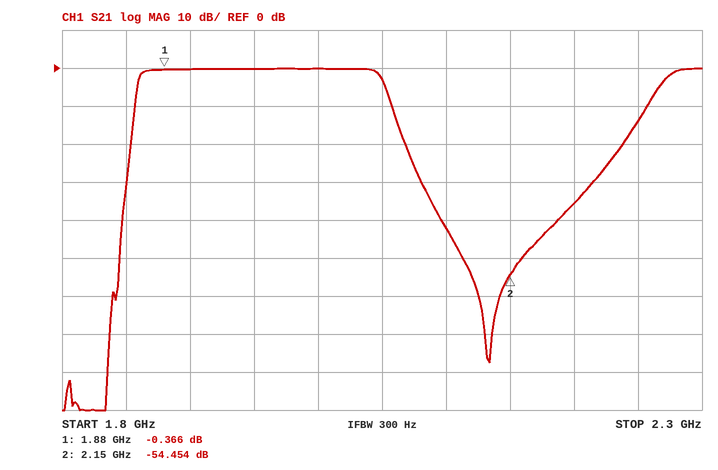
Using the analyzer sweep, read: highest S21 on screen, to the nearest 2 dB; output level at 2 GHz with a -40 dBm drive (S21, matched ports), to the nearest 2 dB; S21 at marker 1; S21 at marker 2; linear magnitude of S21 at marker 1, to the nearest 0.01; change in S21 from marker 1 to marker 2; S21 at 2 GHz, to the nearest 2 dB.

0 dB
-40 dBm
-0.366 dB
-54.454 dB
0.96
-54.088 dB
0 dB
